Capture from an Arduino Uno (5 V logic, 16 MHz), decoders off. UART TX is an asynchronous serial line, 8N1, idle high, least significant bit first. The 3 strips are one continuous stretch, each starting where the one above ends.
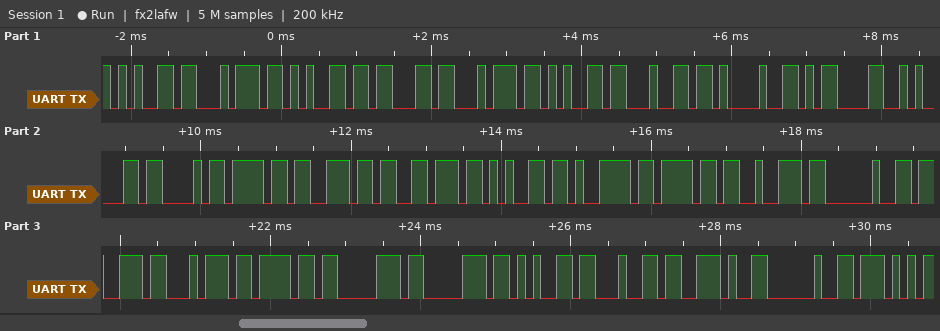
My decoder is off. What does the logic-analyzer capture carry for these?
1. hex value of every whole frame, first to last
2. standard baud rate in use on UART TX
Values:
65 74 65 63 74 65 64 21 0D 0A 43 6F 6E 76 65 79 6F 72 20 73 74 6F 70 70 65 64 2E 20 57
9600 baud
